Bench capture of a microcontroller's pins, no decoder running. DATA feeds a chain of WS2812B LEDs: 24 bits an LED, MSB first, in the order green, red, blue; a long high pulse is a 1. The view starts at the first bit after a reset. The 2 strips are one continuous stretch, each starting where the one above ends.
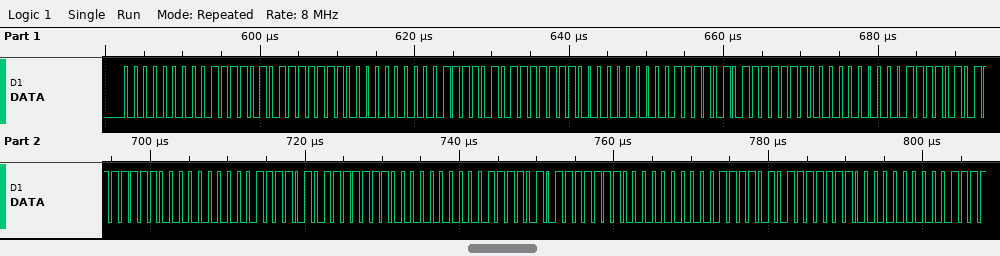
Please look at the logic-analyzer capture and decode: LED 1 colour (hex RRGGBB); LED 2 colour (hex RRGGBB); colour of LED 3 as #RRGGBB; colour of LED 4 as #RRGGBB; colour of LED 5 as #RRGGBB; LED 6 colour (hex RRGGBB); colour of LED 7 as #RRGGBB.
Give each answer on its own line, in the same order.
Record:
#7A00FE
#7A00FE
#7A00FE
#7A00FE
#7A00FE
#7A00FE
#7A00FE
